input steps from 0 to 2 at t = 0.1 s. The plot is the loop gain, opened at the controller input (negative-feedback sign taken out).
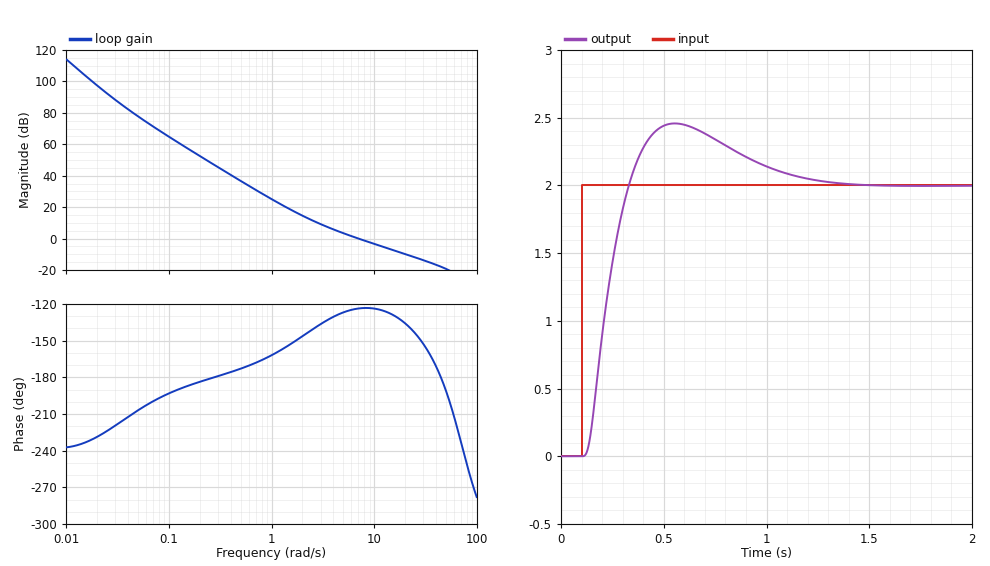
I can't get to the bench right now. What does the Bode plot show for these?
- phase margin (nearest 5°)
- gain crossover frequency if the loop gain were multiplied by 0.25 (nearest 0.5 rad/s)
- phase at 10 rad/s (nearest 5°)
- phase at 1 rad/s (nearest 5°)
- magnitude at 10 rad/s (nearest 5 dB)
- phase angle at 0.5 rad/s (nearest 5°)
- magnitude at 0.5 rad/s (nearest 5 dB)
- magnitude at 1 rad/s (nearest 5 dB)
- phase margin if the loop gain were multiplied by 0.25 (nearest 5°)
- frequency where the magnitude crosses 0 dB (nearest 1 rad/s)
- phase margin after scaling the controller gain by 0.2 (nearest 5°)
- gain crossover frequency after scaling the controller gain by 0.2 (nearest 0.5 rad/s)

55°
2.5 rad/s
-125°
-160°
-5 dB
-175°
35 dB
25 dB
40°
7 rad/s
35°
2.0 rad/s
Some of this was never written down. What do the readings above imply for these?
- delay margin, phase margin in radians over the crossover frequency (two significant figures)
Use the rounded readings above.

0.14 s
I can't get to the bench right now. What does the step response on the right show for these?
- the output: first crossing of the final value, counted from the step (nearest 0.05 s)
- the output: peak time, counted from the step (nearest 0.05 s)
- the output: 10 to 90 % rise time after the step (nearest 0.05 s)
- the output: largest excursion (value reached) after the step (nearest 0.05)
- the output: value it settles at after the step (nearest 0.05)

0.25 s
0.45 s
0.15 s
2.45
2.00
